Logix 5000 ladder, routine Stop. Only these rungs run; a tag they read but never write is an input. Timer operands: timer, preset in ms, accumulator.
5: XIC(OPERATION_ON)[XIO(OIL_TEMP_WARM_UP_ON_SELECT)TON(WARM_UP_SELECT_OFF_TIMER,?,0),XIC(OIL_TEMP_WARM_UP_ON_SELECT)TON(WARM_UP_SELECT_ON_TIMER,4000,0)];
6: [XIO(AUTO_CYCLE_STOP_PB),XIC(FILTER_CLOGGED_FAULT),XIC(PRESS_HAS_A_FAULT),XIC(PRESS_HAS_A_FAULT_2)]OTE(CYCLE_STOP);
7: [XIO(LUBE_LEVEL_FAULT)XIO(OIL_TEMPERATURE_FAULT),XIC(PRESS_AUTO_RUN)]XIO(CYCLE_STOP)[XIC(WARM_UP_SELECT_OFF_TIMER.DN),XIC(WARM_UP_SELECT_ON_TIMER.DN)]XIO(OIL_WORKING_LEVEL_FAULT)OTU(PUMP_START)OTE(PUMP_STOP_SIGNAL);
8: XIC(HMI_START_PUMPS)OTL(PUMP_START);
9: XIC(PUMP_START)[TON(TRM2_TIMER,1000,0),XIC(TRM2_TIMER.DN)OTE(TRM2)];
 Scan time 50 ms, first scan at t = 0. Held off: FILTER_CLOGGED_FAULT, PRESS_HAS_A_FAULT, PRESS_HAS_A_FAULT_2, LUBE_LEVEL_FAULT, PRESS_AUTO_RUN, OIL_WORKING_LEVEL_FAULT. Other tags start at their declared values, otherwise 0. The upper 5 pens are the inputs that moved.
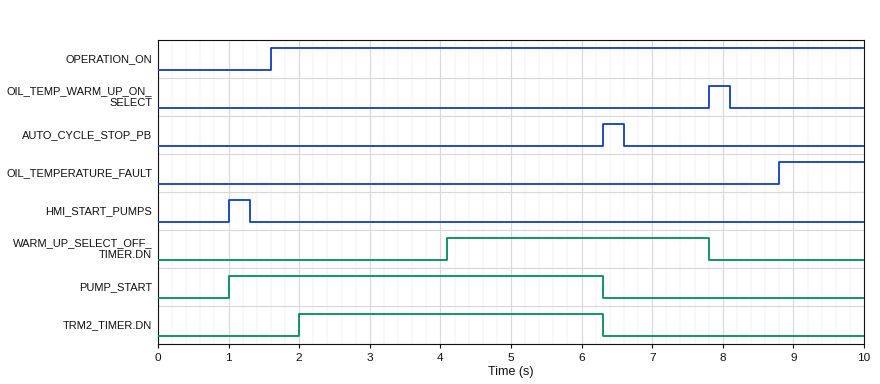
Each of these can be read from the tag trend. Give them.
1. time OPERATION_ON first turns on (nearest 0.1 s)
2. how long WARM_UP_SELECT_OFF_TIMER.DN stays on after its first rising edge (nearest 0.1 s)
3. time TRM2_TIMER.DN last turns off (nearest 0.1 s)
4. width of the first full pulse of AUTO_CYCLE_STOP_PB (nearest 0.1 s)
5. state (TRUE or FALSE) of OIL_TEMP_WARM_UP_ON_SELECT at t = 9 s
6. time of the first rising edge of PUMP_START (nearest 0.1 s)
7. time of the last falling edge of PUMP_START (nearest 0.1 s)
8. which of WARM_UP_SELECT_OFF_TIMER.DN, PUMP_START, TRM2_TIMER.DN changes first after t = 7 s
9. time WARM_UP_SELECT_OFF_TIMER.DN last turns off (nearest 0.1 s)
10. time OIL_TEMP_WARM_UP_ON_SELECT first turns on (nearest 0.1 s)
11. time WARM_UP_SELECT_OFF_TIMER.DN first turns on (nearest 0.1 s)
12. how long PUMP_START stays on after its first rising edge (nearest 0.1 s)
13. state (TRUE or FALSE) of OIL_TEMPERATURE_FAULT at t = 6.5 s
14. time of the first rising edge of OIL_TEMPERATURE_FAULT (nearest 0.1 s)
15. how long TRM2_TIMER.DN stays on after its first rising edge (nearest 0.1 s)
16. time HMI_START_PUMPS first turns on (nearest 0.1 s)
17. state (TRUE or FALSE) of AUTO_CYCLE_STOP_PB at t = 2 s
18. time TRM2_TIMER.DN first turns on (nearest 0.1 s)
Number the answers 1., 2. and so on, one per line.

1. 1.6 s
2. 3.7 s
3. 6.3 s
4. 0.3 s
5. FALSE
6. 1.0 s
7. 6.3 s
8. WARM_UP_SELECT_OFF_TIMER.DN
9. 7.8 s
10. 7.8 s
11. 4.1 s
12. 5.3 s
13. FALSE
14. 8.8 s
15. 4.3 s
16. 1.0 s
17. FALSE
18. 2.0 s
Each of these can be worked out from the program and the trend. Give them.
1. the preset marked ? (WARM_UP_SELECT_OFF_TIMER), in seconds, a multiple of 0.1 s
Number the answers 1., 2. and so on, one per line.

1. 2.5 s
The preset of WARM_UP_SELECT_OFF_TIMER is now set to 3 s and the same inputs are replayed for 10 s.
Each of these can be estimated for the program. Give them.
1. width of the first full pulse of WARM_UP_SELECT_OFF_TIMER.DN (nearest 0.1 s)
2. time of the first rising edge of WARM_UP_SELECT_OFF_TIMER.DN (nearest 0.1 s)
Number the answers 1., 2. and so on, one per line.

1. 3.2 s
2. 4.6 s
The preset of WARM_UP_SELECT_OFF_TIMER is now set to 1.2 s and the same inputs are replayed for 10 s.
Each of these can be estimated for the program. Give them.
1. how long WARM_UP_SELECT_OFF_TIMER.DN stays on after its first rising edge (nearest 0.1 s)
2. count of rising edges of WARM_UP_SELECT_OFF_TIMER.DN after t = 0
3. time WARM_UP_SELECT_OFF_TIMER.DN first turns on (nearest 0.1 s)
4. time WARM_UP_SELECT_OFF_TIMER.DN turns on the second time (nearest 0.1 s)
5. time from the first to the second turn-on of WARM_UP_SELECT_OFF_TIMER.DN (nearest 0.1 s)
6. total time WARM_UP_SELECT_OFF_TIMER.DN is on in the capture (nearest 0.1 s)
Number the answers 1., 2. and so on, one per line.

1. 5.0 s
2. 2
3. 2.8 s
4. 9.3 s
5. 6.5 s
6. 5.7 s
